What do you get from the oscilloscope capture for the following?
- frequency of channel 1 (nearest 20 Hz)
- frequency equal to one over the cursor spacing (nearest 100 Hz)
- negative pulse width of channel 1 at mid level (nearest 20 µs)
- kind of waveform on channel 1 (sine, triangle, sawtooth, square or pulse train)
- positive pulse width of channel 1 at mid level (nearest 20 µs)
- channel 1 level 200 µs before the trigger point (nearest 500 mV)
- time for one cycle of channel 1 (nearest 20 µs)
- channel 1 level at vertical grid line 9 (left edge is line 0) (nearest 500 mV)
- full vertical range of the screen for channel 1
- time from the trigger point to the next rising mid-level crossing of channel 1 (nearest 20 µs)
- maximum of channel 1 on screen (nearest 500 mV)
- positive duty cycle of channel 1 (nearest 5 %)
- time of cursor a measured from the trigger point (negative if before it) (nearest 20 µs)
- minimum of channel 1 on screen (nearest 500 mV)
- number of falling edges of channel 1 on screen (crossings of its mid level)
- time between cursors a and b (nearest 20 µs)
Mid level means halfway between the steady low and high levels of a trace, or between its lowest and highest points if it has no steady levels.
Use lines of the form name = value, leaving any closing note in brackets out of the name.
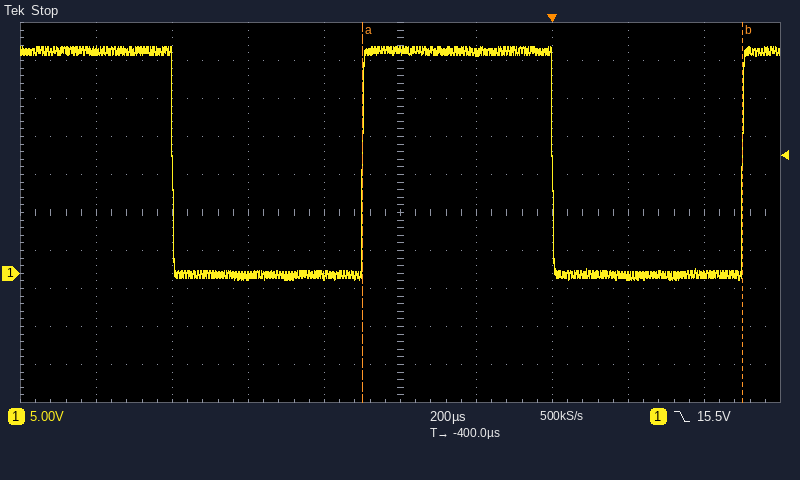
frequency of channel 1 = 1.00 kHz
frequency equal to one over the cursor spacing = 1.0 kHz
negative pulse width of channel 1 at mid level = 500 µs
kind of waveform on channel 1 = square
positive pulse width of channel 1 at mid level = 500 µs
channel 1 level 200 µs before the trigger point = 29.0 V
time for one cycle of channel 1 = 1.00 ms
channel 1 level at vertical grid line 9 (left edge is line 0) = 0.0 V
full vertical range of the screen for channel 1 = 50 V
time from the trigger point to the next rising mid-level crossing of channel 1 = 500 µs
maximum of channel 1 on screen = 30.0 V
positive duty cycle of channel 1 = 50 %
time of cursor a measured from the trigger point (negative if before it) = -500 µs
minimum of channel 1 on screen = -1.0 V
number of falling edges of channel 1 on screen = 2
time between cursors a and b = 1.00 ms
